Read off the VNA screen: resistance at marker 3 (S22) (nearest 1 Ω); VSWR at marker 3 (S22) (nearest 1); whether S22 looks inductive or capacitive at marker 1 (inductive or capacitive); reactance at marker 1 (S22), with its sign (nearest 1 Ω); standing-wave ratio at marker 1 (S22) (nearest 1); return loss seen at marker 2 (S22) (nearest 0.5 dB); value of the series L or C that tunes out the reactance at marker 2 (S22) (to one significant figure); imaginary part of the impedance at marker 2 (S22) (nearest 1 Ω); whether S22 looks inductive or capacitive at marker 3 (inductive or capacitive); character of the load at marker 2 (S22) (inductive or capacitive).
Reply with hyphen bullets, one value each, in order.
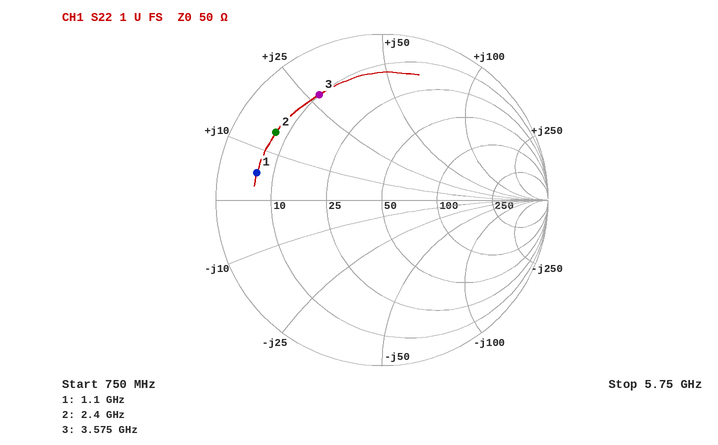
- 10 Ω
- 7
- inductive
- +5 Ω
- 8
- 2.5 dB
- 5 pF
- +14 Ω
- inductive
- inductive
